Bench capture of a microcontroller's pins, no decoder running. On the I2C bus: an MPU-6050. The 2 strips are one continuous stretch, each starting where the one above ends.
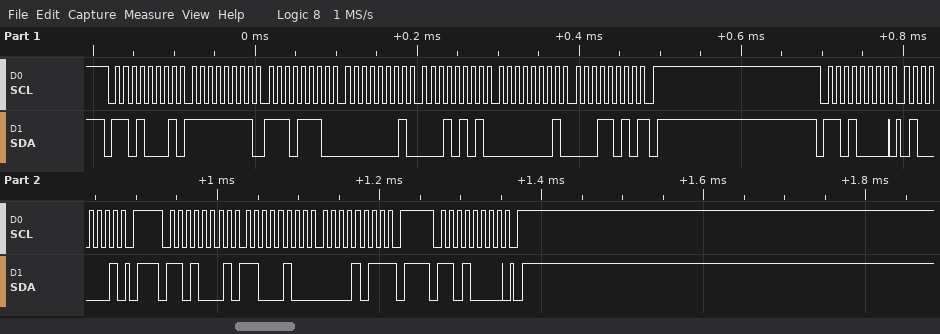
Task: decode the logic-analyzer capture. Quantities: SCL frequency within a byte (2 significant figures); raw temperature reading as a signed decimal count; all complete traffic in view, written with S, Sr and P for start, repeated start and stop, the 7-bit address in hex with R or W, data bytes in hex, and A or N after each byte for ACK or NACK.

100 kHz
-15349
S 68R A FF A EE A 01 A 15 A 01 A 1A N P S 68W A 41 A P S 68R A C4 A 0B N P S 68W A P
